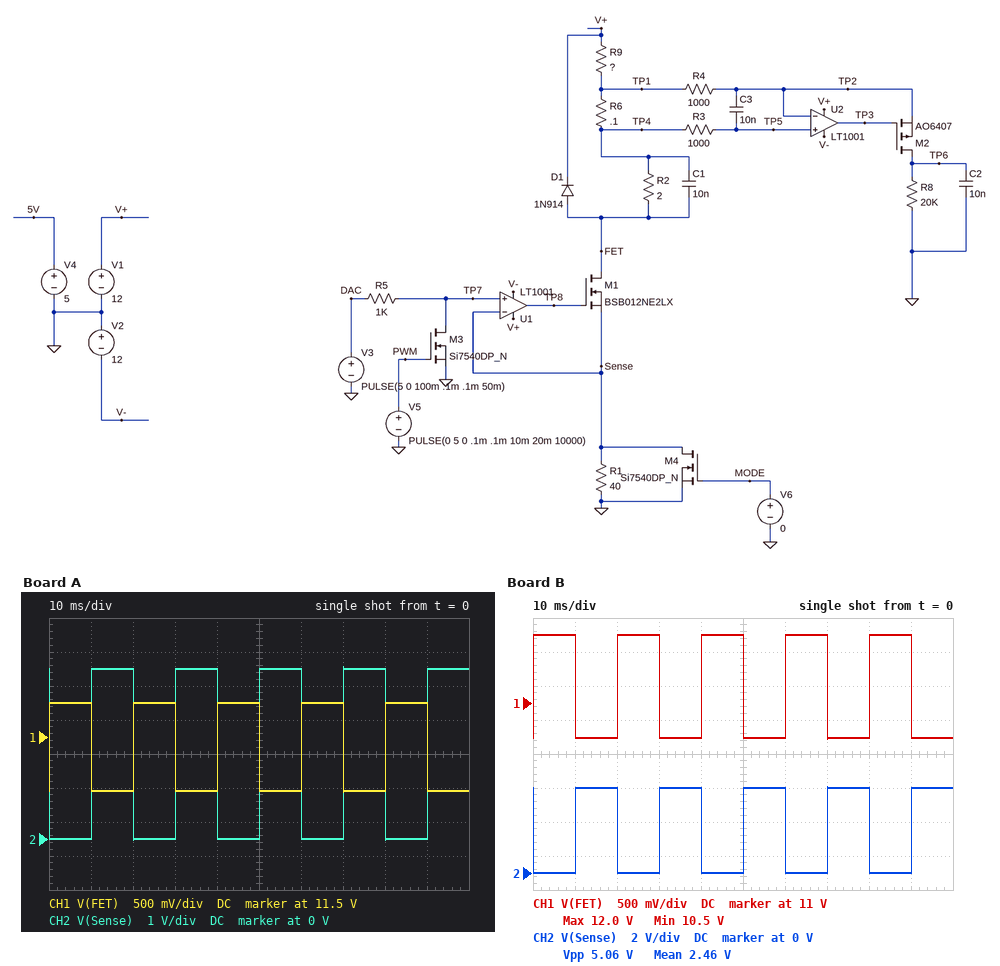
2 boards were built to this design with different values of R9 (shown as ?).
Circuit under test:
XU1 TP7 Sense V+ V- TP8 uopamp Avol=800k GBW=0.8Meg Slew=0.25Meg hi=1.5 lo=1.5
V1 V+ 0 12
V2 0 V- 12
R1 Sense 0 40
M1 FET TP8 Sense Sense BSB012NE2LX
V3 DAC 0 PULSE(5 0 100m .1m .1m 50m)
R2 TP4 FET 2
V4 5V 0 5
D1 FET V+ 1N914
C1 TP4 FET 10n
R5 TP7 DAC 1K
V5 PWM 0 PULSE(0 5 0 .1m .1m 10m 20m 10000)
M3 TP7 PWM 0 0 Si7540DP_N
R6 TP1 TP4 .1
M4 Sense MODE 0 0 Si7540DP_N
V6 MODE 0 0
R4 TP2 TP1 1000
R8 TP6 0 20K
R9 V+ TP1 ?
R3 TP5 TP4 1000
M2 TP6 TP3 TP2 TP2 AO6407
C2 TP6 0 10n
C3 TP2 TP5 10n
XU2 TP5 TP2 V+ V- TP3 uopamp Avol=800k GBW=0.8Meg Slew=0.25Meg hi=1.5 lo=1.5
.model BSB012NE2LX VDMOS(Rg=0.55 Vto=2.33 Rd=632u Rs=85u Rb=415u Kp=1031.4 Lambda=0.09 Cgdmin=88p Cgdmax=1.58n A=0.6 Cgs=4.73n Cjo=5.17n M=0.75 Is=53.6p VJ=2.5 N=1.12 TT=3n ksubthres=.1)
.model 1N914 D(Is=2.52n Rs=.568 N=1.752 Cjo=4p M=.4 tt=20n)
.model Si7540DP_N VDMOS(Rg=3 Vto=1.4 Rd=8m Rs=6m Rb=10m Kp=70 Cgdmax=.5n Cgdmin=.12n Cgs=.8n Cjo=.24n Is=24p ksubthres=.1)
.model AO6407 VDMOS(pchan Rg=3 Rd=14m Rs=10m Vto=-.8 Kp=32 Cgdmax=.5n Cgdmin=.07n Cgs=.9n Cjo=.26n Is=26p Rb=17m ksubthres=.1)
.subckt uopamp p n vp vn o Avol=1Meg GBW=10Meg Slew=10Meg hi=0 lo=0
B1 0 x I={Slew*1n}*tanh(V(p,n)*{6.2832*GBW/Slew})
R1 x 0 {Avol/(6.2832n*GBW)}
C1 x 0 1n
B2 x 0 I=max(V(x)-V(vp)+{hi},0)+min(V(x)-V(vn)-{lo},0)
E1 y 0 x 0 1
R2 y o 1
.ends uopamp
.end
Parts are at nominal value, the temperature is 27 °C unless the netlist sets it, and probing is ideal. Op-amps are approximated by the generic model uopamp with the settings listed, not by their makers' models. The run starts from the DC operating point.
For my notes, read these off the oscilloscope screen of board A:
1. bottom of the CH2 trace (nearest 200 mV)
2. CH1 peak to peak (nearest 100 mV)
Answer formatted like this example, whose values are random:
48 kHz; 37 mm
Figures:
0 V; 1.3 V
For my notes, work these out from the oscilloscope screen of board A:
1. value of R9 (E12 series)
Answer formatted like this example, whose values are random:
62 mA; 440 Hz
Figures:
8.2 Ω
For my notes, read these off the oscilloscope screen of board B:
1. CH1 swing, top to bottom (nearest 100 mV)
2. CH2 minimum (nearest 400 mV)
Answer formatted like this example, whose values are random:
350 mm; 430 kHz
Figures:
1.5 V; 0 V
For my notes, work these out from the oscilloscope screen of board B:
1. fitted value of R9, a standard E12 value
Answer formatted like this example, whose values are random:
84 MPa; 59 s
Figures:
10 Ω
